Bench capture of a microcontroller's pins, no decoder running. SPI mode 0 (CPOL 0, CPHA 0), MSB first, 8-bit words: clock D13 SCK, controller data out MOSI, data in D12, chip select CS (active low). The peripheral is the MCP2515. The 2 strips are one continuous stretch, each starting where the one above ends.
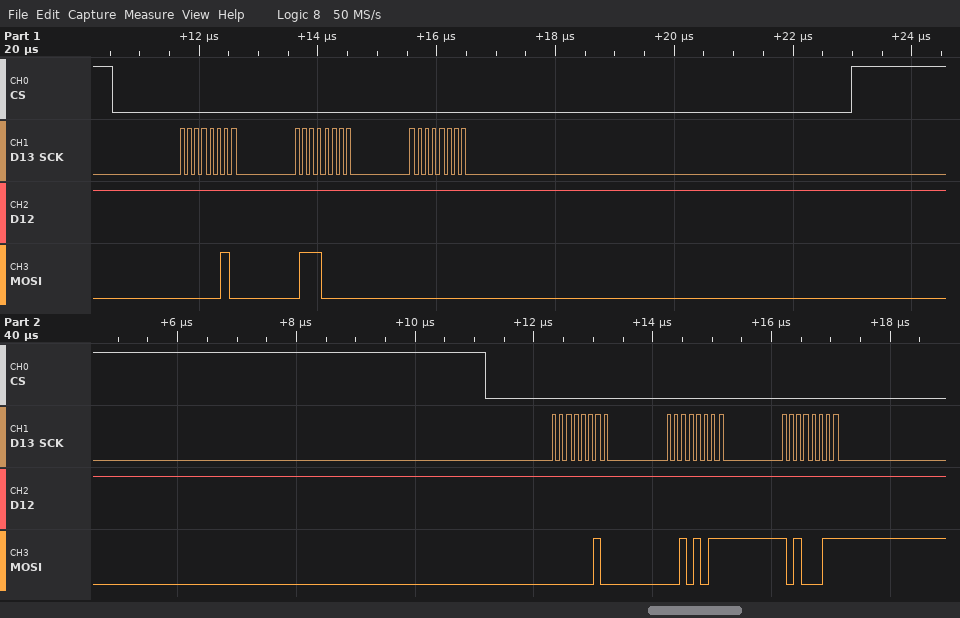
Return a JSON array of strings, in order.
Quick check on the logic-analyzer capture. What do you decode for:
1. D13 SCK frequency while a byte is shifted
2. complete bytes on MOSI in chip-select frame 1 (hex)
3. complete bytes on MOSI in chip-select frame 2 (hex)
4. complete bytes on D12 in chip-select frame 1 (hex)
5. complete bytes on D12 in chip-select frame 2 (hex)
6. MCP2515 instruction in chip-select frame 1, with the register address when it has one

["8 MHz", "02 70 00", "02 2B A3", "FF FF FF", "FF FF FF", "WRITE 0x70"]
